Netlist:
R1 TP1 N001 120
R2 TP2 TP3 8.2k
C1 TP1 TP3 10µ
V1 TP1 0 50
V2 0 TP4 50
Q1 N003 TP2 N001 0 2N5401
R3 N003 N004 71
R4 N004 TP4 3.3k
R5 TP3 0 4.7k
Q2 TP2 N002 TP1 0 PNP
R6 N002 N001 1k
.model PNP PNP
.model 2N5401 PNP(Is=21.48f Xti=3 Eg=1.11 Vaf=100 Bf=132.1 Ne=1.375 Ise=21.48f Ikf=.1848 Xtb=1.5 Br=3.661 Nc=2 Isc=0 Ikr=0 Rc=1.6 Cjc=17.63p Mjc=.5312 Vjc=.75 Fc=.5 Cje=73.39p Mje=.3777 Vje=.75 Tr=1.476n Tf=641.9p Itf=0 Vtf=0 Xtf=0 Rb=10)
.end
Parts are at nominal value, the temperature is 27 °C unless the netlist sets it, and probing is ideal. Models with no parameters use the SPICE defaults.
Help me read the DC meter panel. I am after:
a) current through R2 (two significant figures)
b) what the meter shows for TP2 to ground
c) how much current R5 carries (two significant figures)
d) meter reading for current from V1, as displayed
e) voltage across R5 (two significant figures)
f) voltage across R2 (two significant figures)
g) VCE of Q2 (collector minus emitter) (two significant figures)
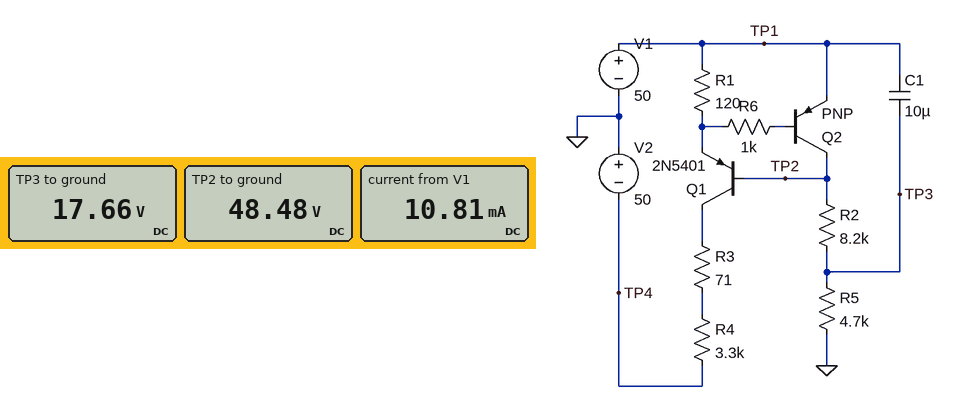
3.8 mA
48.48 V
3.8 mA
10.81 mA
18 V
31 V
-1.5 V
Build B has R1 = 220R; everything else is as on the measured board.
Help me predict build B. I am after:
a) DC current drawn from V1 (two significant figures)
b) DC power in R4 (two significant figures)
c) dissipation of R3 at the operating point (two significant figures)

7.6 mA
49 mW
1.1 mW
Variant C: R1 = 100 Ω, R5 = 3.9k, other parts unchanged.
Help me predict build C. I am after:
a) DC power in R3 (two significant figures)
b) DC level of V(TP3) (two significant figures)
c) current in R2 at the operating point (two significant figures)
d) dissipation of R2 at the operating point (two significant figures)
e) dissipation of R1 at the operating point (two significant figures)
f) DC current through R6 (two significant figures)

5.1 mW
16 V
4.0 mA
130 mW
7.2 mW
40 µA
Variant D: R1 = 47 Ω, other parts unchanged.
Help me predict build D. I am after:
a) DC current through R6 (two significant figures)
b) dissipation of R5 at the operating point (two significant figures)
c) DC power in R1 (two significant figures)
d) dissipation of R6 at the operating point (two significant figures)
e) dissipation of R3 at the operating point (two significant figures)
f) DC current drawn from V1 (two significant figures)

36 µA
66 mW
15 mW
1.3 µW
23 mW
22 mA
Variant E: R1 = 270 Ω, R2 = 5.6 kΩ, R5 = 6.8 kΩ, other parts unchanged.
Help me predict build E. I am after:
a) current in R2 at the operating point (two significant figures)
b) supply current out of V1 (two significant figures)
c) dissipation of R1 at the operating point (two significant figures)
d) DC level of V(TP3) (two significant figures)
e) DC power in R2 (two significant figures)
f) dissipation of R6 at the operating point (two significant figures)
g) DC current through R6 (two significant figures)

3.9 mA
7.1 mA
2.7 mW
27 V
86 mW
1.5 µW
39 µA
